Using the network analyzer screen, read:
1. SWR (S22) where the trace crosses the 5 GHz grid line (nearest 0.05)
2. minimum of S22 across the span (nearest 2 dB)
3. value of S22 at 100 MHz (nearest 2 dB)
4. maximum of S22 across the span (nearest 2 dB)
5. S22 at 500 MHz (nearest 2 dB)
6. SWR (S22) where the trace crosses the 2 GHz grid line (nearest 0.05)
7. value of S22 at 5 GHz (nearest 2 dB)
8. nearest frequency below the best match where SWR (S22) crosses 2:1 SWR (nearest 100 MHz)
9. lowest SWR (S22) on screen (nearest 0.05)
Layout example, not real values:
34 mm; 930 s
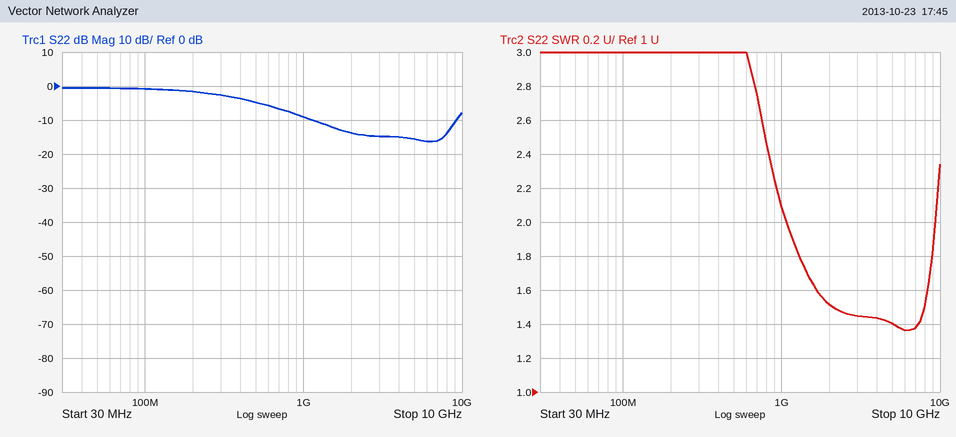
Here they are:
1.40; -16 dB; 0 dB; 0 dB; -4 dB; 1.50; -16 dB; 1.1 GHz; 1.35
